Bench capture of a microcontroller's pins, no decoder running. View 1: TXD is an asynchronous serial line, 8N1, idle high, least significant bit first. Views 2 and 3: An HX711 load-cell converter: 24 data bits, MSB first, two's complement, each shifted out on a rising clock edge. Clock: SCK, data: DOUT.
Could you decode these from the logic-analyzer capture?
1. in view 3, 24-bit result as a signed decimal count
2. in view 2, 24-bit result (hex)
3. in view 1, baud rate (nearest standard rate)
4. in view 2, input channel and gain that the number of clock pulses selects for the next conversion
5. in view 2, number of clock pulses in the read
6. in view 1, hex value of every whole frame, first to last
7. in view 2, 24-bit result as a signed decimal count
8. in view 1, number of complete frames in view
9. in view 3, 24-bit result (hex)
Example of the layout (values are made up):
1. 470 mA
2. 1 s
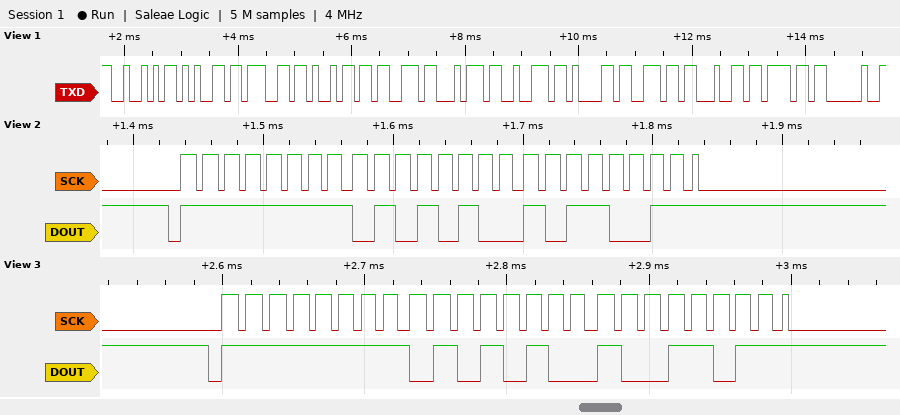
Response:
1. -43877
2. 0xFF54B3
3. 9600 baud
4. channel A, gain 128
5. 25
6. 52 65 67 69 73 74 72 61 6E 64 6F 20
7. -43853
8. 12
9. 0xFF549B
